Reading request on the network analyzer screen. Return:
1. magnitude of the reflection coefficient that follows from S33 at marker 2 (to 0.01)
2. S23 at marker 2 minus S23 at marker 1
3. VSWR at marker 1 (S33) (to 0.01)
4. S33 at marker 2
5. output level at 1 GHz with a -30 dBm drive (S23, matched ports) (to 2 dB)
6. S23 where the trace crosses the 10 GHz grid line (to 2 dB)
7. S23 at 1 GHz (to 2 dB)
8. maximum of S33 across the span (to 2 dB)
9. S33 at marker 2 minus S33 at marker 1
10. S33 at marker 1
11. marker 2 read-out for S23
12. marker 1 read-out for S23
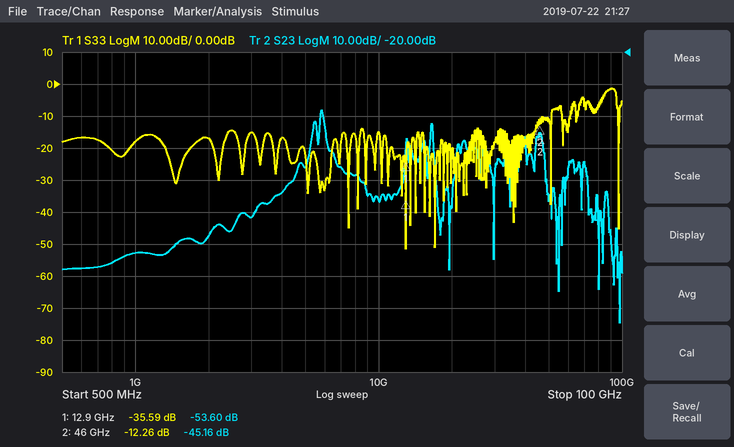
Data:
0.24
8.44 dB
1.03
-12.26 dB
-112 dBm
-66 dB
-82 dB
-2 dB
23.33 dB
-35.59 dB
-45.16 dB
-53.60 dB
